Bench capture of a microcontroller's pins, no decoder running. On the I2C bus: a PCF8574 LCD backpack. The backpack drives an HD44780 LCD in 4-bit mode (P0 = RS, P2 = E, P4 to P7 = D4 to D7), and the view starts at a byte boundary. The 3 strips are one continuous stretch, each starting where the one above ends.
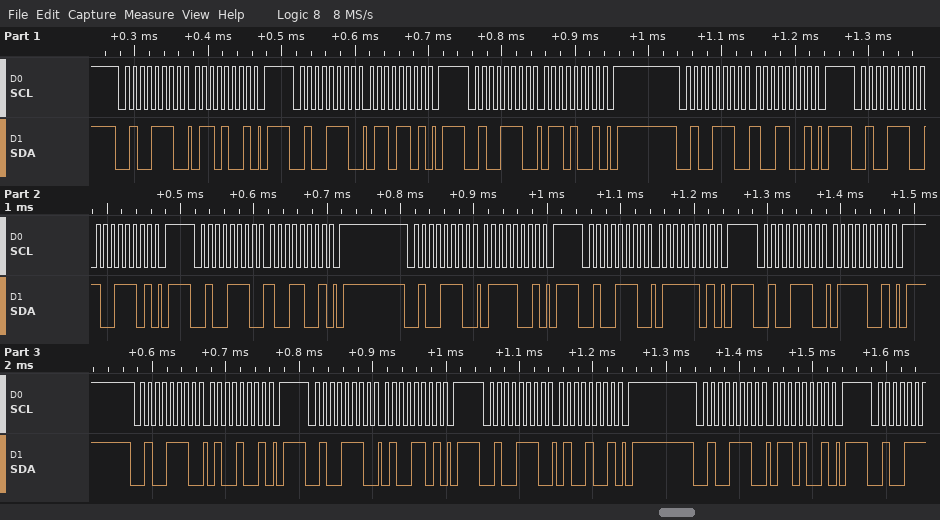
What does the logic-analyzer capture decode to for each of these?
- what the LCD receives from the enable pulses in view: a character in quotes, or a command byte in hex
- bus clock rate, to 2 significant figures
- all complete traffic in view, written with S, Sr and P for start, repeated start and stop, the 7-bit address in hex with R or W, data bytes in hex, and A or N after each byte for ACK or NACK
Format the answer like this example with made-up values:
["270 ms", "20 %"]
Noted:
["'i' 't'", "100 kHz", "S 27W A 69 A P S 27W A 6D A P S 27W A 69 A P S 27W A 99 A P S 27W A 9D A P S 27W A 99 A P S 27W A 79 A P S 27W A 7D A P S 27W A 79 A P S 27W A 49 A P S 27W A 4D A P S 27W A 49 A P S 27W A 69 A P"]
